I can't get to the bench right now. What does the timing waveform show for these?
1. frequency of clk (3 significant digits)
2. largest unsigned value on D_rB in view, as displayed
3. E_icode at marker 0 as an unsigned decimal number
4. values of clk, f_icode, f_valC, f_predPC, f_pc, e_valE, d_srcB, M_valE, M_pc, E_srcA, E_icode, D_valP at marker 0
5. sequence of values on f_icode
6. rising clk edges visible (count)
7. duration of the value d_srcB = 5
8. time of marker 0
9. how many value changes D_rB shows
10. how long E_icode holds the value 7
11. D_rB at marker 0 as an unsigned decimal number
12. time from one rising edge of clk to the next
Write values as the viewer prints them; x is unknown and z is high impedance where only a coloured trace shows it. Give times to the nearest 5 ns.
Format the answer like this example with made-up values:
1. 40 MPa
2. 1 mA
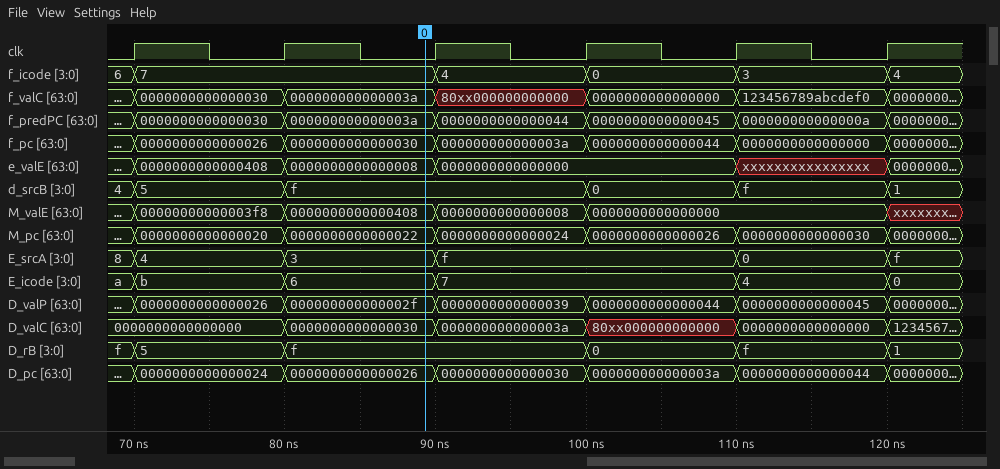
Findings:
1. 100 MHz
2. f
3. 6
4. clk=0, f_icode=7, f_valC=000000000000003a, f_predPC=000000000000003a, f_pc=0000000000000030, e_valE=0000000000000008, d_srcB=f, M_valE=0000000000000408, M_pc=0000000000000022, E_srcA=3, E_icode=6, D_valP=000000000000002f
5. 6, 7, 4, 0, 3, 4
6. 6
7. 10 ns
8. 90 ns
9. 5
10. 20 ns
11. 15
12. 10 ns
